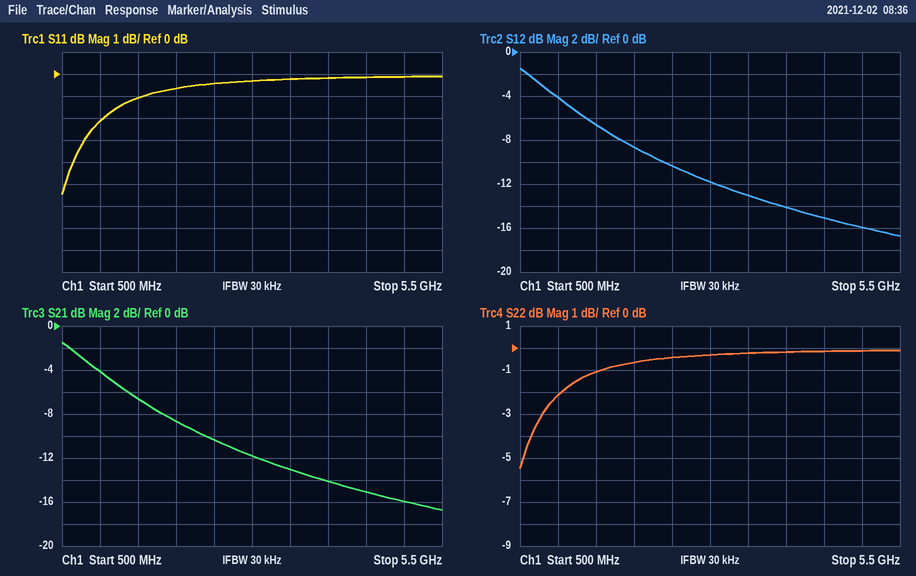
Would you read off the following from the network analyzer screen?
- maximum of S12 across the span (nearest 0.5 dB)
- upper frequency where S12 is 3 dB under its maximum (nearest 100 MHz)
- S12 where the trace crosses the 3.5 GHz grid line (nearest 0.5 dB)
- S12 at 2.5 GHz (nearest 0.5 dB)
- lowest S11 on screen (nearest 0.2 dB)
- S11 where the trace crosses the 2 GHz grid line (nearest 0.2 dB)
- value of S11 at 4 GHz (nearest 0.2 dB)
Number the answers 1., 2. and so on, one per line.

1. -1.5 dB
2. 1.1 GHz
3. -13.0 dB
4. -10.5 dB
5. -5.4 dB
6. -0.6 dB
7. -0.2 dB
